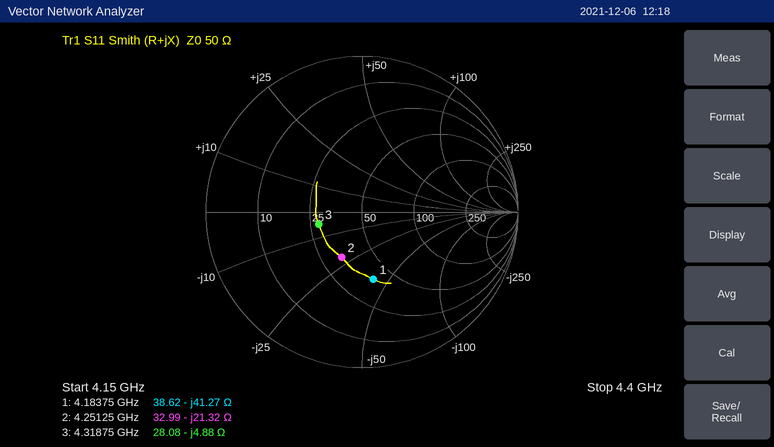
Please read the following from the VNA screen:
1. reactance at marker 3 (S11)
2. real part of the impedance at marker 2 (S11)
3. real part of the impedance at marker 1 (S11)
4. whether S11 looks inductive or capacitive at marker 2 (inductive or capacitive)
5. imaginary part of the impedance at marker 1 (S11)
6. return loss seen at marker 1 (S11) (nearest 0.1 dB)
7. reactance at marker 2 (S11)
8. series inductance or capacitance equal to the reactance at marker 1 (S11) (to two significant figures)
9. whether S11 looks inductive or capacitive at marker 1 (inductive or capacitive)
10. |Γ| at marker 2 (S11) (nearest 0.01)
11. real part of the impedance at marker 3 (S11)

-4.88 Ω
32.99 Ω
38.62 Ω
capacitive
-41.27 Ω
7.2 dB
-21.32 Ω
920 fF
capacitive
0.32
28.08 Ω
